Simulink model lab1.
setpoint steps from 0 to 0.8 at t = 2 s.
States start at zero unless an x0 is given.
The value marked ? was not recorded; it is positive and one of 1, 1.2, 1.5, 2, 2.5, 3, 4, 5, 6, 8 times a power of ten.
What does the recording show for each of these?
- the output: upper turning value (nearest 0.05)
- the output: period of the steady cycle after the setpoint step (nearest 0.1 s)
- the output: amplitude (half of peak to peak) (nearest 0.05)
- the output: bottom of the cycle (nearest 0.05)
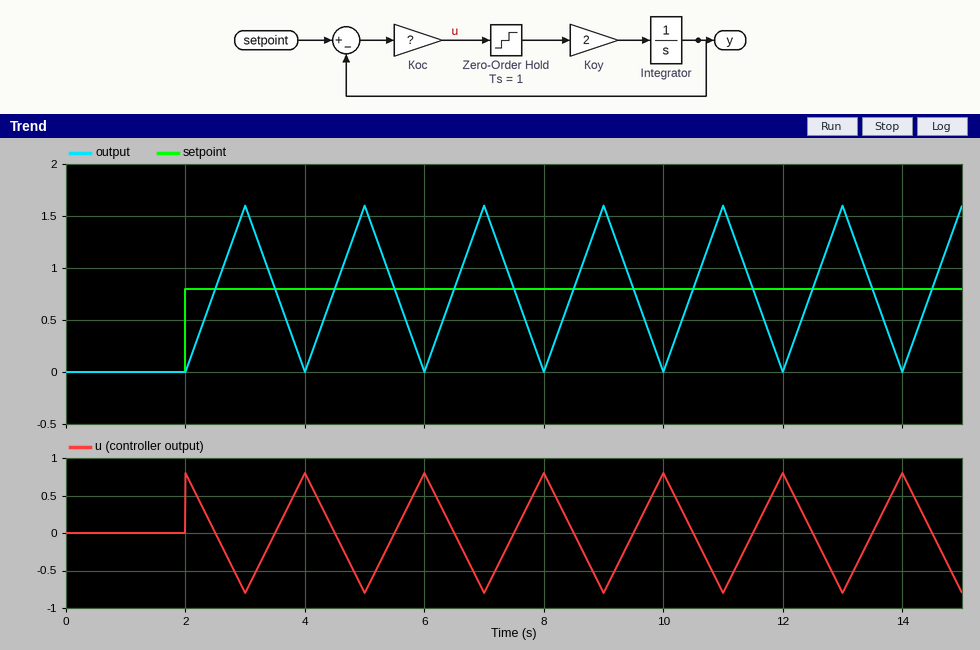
1.60
2.0 s
0.80
0.00
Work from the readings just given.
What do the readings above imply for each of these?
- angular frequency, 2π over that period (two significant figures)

3.1 rad/s
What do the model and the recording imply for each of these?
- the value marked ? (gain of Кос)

1
